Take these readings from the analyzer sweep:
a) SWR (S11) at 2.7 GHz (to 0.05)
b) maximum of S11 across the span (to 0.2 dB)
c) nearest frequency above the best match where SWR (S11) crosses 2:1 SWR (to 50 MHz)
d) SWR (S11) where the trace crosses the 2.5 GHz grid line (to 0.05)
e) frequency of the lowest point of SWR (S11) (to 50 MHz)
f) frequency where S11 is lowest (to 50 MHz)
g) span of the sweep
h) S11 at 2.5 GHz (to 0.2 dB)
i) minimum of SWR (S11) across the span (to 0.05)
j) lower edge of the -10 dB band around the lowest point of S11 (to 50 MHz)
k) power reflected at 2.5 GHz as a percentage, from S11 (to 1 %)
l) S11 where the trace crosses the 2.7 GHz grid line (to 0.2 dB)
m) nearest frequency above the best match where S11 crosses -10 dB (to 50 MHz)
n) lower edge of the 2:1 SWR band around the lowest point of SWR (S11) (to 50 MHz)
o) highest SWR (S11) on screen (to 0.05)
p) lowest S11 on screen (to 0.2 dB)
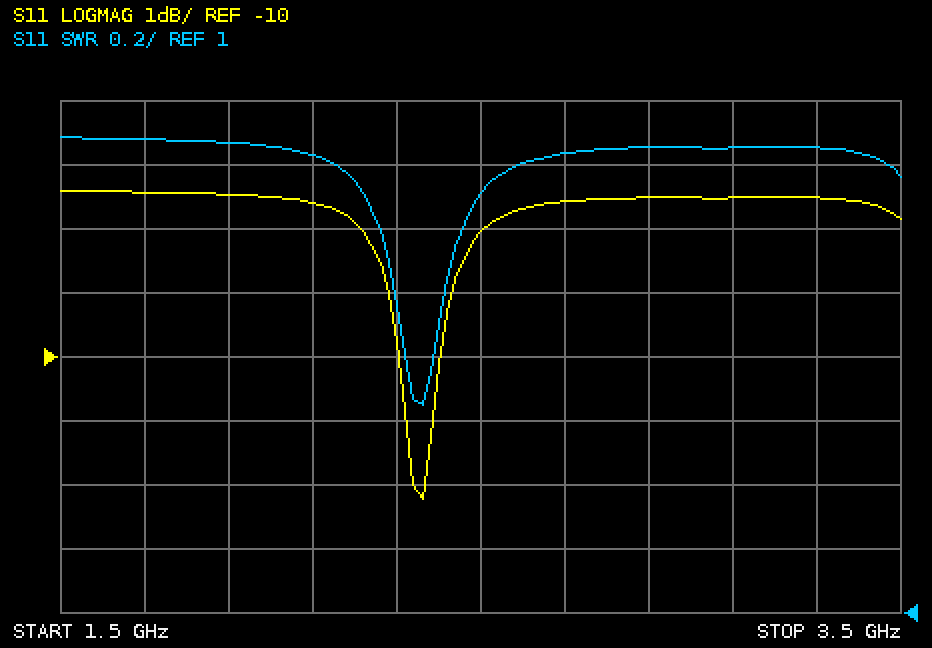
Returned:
2.45
-7.4 dB
2.40 GHz
2.30
2.35 GHz
2.35 GHz
2 GHz
-8.0 dB
1.65
2.30 GHz
16 %
-7.6 dB
2.40 GHz
2.30 GHz
2.50
-12.2 dB
